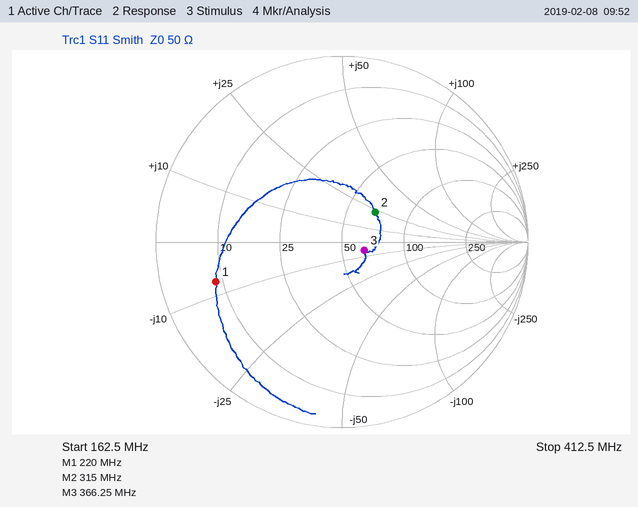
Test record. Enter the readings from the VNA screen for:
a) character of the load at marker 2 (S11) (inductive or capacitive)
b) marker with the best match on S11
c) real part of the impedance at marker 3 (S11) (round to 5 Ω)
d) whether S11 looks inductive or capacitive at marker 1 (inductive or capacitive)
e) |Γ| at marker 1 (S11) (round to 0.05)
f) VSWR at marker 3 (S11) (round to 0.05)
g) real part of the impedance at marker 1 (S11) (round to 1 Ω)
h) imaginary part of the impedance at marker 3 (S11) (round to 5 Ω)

inductive
marker 3
65 Ω
capacitive
0.70
1.30
9 Ω
-5 Ω
